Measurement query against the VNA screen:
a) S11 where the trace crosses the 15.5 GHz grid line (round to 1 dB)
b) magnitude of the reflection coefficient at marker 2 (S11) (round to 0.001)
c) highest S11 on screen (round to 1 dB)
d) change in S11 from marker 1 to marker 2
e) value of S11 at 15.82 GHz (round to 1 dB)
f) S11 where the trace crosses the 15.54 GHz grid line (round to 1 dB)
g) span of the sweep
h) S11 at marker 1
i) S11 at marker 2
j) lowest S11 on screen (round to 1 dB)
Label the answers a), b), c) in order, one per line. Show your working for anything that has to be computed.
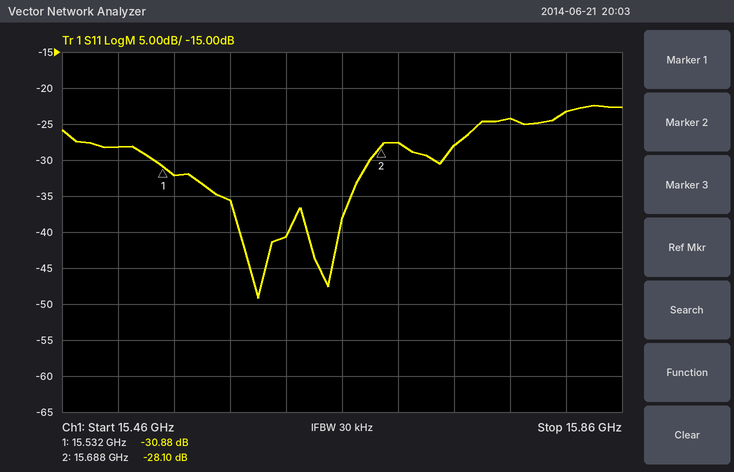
a) -28 dB
b) 10^(-28.1/20) ≈ 0.039
c) -22 dB
d) -28.1 − (-30.88) = 2.78 dB
e) -23 dB
f) -32 dB
g) 400 MHz
h) -30.88 dB
i) -28.10 dB
j) -49 dB
